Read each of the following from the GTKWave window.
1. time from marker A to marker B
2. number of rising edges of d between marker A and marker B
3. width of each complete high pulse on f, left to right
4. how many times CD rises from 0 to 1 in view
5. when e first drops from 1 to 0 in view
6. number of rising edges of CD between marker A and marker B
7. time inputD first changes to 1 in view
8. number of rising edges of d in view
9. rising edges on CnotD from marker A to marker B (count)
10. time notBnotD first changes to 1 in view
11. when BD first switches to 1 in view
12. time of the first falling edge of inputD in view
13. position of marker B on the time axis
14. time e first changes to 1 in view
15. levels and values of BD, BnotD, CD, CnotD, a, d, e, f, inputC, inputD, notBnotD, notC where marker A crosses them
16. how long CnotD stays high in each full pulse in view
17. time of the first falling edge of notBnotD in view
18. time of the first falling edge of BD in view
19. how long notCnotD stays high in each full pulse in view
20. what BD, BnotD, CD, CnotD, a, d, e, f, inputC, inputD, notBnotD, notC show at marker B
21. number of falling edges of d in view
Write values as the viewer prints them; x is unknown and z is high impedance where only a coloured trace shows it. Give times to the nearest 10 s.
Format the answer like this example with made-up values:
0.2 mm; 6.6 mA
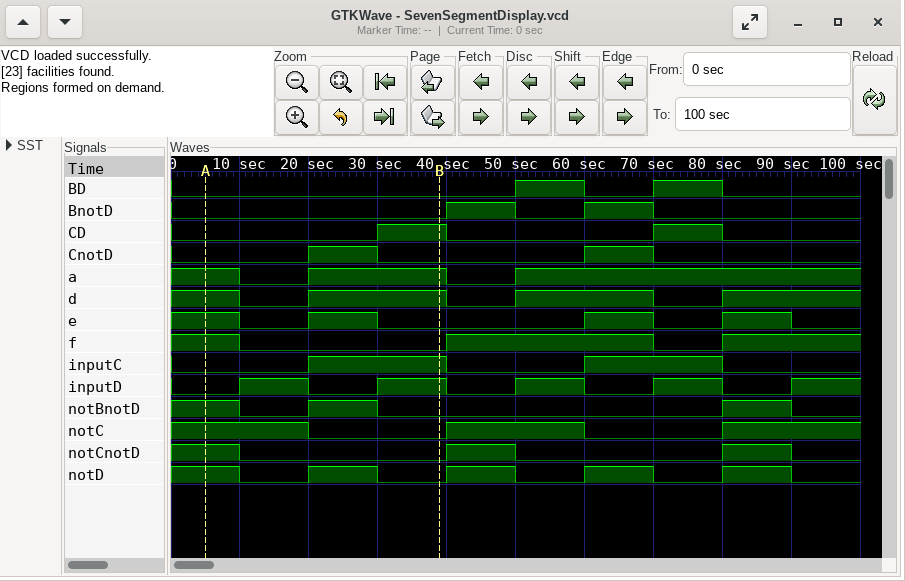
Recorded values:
30 s; 1; 30 s; 2; 10 s; 1; 10 s; 3; 1; 20 s; 50 s; 20 s; 40 s; 20 s; BD=0, BnotD=0, CD=0, CnotD=0, a=1, d=1, e=1, f=1, inputC=0, inputD=0, notBnotD=1, notC=1; 10 s, 10 s; 10 s; 60 s; 10 s, 10 s; BD=0, BnotD=0, CD=1, CnotD=0, a=1, d=1, e=0, f=0, inputC=1, inputD=1, notBnotD=0, notC=0; 3
